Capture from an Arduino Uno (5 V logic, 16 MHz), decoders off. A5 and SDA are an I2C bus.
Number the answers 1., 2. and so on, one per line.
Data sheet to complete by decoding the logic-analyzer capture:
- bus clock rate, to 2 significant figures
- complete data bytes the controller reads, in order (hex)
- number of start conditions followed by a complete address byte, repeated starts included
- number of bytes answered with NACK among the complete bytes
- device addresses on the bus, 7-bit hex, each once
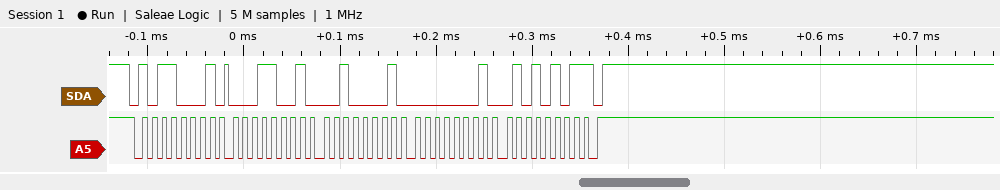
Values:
1. 100 kHz
2. 19 21 01 55
3. 1
4. 1
5. 0x58
